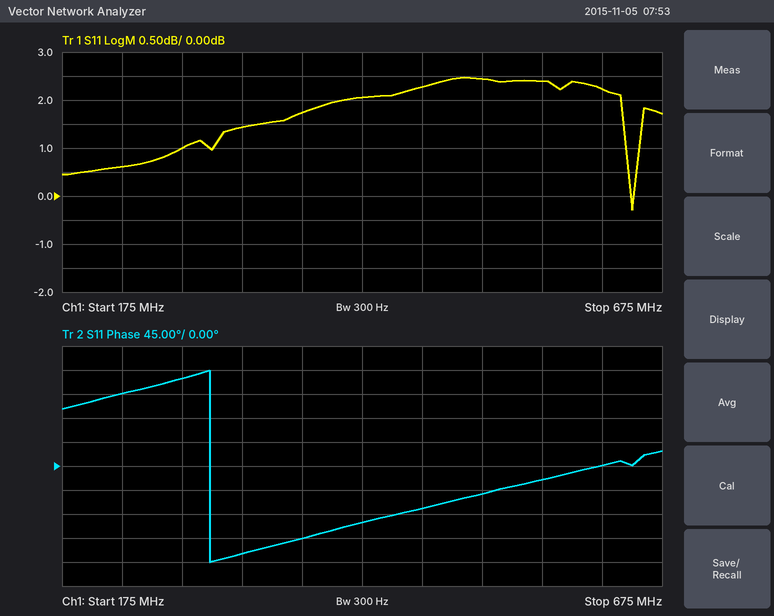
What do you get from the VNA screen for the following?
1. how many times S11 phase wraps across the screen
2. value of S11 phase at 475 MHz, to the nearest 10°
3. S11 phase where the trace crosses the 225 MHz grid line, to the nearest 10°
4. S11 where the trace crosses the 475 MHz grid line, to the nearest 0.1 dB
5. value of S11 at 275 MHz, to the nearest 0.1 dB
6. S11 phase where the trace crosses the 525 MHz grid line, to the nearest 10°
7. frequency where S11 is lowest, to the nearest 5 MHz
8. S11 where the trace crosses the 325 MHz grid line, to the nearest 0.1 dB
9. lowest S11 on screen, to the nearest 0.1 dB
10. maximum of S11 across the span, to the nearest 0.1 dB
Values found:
1
-80°
140°
2.3 dB
1.0 dB
-50°
650 MHz
1.4 dB
-0.3 dB
2.5 dB
